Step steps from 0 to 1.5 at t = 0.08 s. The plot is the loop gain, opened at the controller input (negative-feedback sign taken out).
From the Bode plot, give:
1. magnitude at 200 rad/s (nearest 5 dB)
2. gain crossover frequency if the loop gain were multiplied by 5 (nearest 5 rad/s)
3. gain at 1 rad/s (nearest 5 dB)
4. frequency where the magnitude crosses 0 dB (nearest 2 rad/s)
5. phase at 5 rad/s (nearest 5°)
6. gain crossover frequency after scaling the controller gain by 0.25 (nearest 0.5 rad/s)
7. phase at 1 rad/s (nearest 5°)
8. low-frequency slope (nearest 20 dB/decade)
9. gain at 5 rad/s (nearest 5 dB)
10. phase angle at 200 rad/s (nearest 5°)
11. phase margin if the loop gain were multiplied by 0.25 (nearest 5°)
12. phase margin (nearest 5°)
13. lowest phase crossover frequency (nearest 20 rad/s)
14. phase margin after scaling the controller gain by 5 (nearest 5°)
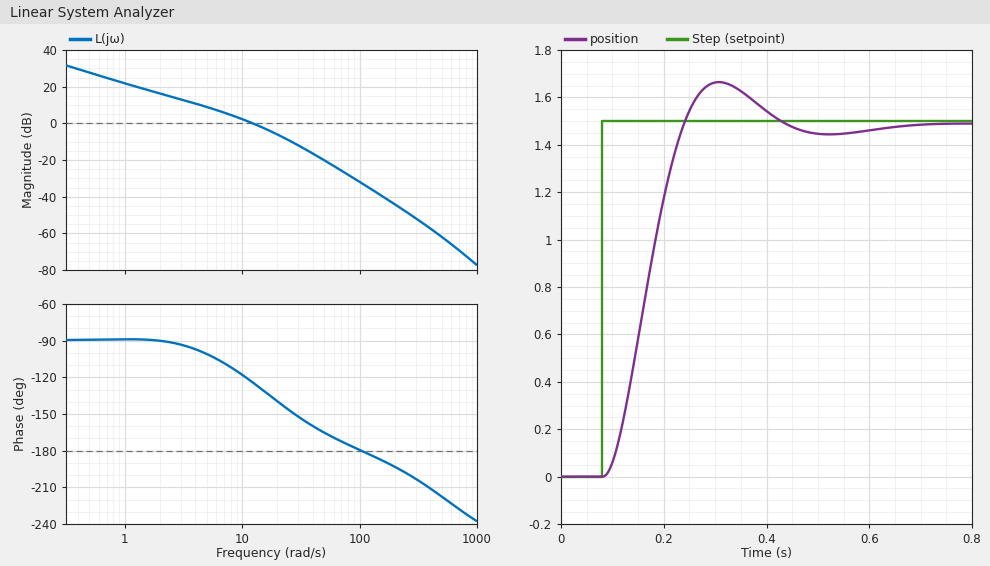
-45 dB
35 rad/s
20 dB
12 rad/s
-100°
3.5 rad/s
-90°
-20 dB/decade
10 dB
-195°
85°
55°
100 rad/s
25°
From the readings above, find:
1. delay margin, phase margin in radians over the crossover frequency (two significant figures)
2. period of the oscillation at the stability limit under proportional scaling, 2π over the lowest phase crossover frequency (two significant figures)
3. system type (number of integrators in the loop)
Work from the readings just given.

0.080 s
0.063 s
1
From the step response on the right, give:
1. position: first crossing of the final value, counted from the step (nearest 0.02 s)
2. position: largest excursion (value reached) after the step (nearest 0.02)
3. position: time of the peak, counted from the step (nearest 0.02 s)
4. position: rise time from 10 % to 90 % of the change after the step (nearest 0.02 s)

0.16 s
1.66
0.22 s
0.10 s
